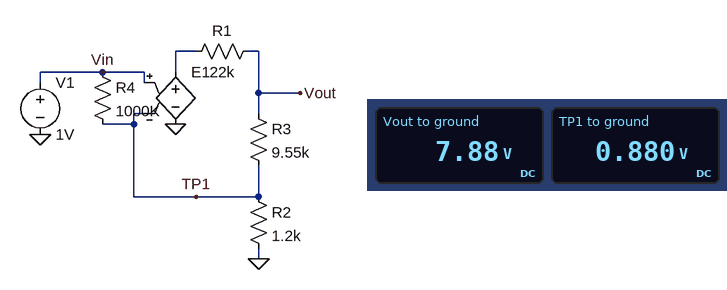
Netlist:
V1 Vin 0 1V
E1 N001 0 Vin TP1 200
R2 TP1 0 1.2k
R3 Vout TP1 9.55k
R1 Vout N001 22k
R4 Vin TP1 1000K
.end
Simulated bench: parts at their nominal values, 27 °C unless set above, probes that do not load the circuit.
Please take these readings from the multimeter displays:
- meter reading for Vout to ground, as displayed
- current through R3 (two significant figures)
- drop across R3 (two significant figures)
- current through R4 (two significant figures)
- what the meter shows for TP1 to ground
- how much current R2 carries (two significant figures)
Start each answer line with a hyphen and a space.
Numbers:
- 7.88 V
- 730 µA
- 7.0 V
- 120 nA
- 0.880 V
- 730 µA
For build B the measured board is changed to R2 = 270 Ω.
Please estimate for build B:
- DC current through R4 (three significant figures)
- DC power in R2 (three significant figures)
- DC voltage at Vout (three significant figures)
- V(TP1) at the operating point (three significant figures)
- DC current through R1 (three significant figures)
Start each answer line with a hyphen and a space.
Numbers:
- 371 nA
- 1.47 mW
- 22.9 V
- 629 mV
- 2.33 mA
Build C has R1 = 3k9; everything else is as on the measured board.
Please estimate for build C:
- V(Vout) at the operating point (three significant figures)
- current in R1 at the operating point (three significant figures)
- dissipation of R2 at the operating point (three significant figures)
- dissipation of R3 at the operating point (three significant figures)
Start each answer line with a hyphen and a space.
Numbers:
- 8.44 V
- 785 µA
- 740 µW
- 5.89 mW
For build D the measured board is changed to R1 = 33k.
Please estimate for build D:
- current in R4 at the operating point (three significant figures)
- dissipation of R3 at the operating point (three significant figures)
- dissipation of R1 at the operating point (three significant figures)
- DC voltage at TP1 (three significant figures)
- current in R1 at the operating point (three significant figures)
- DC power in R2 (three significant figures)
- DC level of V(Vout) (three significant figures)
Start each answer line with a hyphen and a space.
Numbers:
- 154 nA
- 4.74 mW
- 16.4 mW
- 846 mV
- 705 µA
- 596 µW
- 7.58 V
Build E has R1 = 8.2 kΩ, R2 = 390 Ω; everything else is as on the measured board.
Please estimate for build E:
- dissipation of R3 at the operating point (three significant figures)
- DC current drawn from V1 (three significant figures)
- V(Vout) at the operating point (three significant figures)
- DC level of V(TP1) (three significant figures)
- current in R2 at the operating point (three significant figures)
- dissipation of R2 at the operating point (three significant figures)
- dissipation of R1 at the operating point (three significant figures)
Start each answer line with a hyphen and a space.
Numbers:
- 41.3 mW
- 189 nA
- 20.7 V
- 811 mV
- 2.08 mA
- 1.69 mW
- 35.5 mW
